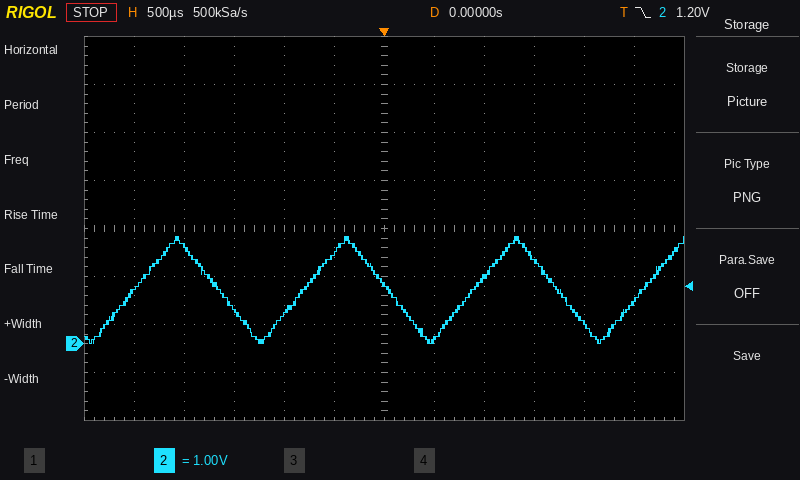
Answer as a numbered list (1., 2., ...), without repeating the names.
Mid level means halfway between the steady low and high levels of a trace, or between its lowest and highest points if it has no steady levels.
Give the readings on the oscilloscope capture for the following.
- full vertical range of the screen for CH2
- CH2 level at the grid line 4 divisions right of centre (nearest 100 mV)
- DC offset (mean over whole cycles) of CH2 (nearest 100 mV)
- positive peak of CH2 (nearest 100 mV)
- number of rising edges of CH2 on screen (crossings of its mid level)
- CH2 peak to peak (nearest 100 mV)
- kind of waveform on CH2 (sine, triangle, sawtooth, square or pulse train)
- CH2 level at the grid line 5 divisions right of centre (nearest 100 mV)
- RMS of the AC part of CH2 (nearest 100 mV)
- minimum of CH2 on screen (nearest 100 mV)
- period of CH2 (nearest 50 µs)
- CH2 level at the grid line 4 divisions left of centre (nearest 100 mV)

1. 8 V
2. 400 mV
3. 1.1 V
4. 2.2 V
5. 4
6. 2.2 V
7. triangle
8. 900 mV
9. 600 mV
10. 0.0 V
11. 1.70 ms
12. 2.0 V
